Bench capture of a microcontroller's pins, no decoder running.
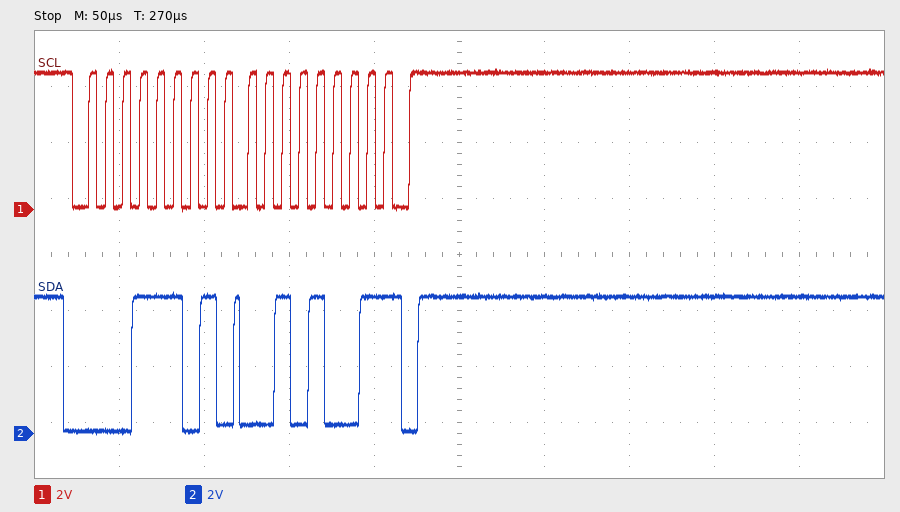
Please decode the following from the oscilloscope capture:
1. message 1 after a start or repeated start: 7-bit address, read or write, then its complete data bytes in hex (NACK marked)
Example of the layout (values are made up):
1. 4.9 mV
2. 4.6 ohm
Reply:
1. 0x0E read: 29 NACK
